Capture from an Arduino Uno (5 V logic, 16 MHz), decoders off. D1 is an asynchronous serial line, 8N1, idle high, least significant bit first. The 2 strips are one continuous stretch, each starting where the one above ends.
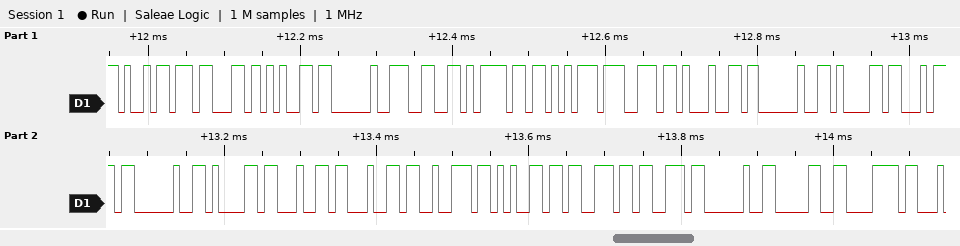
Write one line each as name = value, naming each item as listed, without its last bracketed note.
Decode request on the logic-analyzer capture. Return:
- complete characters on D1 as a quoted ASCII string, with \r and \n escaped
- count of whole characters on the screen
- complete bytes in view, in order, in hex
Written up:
complete characters on D1 as a quoted ASCII string, with \r and \n escaped = "ice found at address 0x"
count of whole characters on the screen = 23
complete bytes in view, in order, in hex = 69 63 65 20 66 6F 75 6E 64 20 61 74 20 61 64 64 72 65 73 73 20 30 78
